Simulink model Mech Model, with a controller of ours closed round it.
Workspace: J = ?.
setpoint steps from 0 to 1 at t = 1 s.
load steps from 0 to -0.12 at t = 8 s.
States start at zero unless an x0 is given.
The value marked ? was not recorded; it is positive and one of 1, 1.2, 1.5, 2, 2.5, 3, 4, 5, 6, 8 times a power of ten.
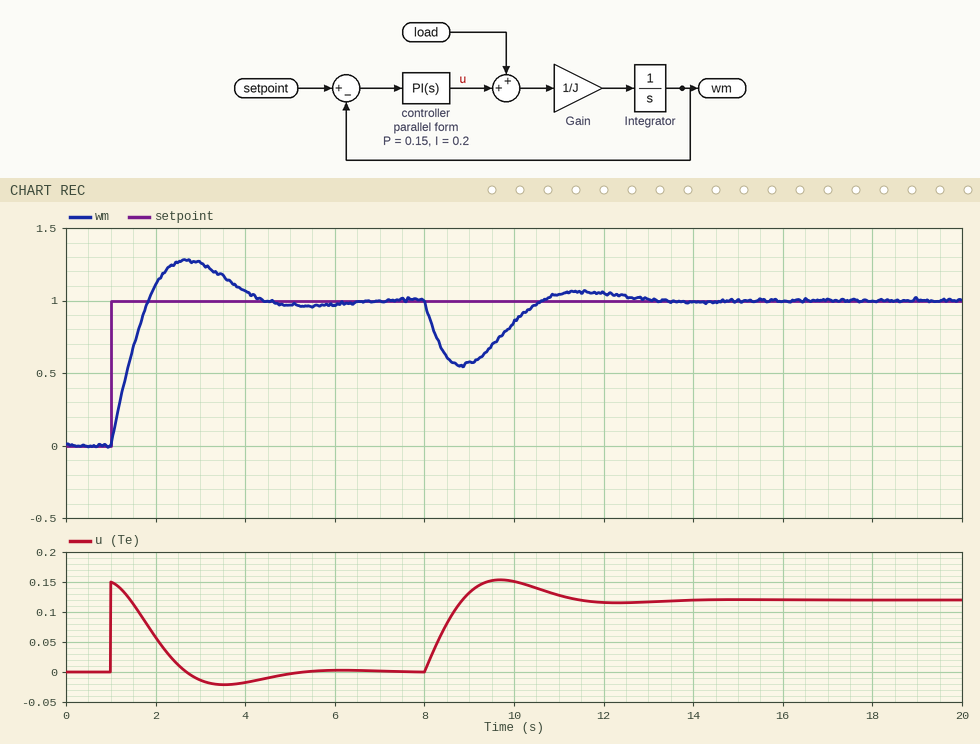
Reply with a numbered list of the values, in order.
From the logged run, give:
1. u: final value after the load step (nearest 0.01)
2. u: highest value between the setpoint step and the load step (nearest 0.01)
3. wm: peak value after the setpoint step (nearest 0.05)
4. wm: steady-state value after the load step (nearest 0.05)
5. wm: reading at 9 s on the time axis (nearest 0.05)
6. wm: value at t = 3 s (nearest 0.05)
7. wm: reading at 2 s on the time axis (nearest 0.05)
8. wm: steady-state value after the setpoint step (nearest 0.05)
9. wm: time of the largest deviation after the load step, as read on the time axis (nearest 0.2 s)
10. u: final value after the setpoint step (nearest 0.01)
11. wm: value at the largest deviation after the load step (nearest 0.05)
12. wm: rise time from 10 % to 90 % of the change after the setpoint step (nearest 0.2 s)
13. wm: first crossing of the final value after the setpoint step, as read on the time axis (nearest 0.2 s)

1. 0.12
2. 0.15
3. 1.30
4. 1.00
5. 0.55
6. 1.25
7. 1.10
8. 1.00
9. 8.8 s
10. 0.00
11. 0.55
12. 0.6 s
13. 1.8 s
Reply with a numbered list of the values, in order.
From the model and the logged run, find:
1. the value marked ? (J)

1. 0.1
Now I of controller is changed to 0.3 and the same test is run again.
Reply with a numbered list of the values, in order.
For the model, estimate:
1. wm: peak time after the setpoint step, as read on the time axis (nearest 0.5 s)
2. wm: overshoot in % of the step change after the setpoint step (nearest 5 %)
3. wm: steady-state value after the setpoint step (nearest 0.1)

1. 2.5 s
2. 35 %
3. 1.0
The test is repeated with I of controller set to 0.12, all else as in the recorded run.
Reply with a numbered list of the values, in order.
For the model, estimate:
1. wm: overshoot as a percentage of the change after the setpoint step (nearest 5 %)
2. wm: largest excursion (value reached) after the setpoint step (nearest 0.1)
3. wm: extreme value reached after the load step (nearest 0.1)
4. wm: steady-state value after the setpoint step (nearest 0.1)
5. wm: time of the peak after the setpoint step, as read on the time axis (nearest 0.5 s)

1. 20 %
2. 1.2
3. 0.5
4. 1.0
5. 3.0 s
